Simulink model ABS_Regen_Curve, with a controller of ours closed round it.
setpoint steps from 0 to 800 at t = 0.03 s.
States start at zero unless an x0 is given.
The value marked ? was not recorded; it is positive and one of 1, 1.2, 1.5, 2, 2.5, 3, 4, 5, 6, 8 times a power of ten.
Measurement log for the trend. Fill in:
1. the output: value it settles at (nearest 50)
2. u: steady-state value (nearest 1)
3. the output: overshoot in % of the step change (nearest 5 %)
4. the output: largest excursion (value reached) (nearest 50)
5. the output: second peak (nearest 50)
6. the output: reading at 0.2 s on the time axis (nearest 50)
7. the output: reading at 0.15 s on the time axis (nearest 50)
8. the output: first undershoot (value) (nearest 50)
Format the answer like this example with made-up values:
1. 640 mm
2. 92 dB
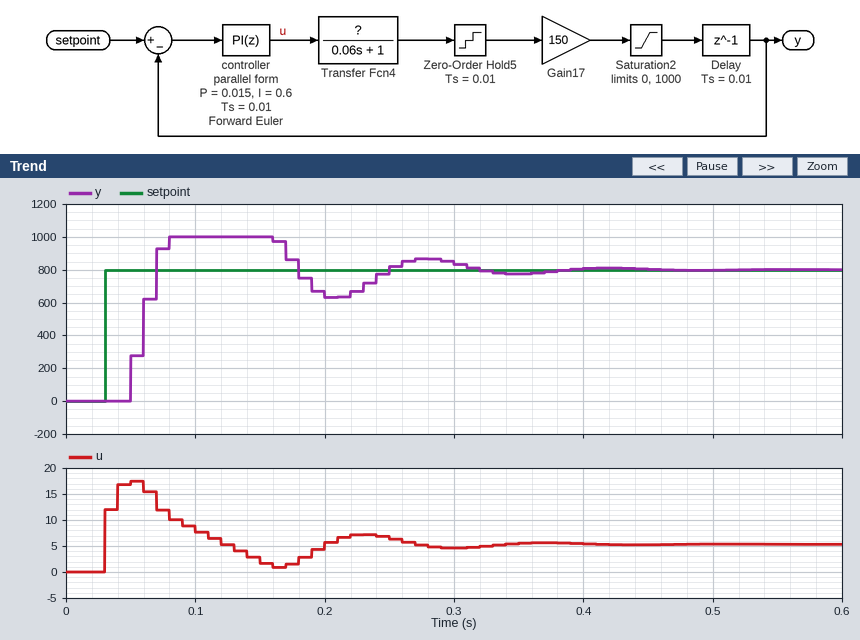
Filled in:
1. 800
2. 5
3. 25 %
4. 1000
5. 850
6. 650
7. 1000
8. 650
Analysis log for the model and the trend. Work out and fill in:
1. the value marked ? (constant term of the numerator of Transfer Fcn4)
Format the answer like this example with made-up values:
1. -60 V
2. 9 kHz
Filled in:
1. 1
